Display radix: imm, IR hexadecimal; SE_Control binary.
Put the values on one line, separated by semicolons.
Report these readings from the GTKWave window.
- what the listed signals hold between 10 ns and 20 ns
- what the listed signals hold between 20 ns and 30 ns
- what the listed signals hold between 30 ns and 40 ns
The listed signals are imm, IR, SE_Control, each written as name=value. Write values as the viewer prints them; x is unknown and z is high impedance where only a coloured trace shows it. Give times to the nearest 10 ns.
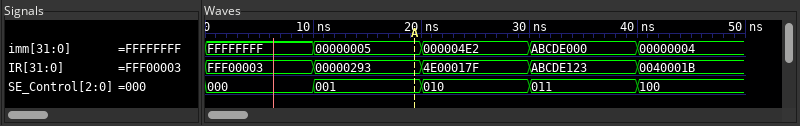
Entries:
imm=00000005, IR=00000293, SE_Control=001; imm=000004E2, IR=4E00017F, SE_Control=010; imm=ABCDE000, IR=ABCDE123, SE_Control=011
